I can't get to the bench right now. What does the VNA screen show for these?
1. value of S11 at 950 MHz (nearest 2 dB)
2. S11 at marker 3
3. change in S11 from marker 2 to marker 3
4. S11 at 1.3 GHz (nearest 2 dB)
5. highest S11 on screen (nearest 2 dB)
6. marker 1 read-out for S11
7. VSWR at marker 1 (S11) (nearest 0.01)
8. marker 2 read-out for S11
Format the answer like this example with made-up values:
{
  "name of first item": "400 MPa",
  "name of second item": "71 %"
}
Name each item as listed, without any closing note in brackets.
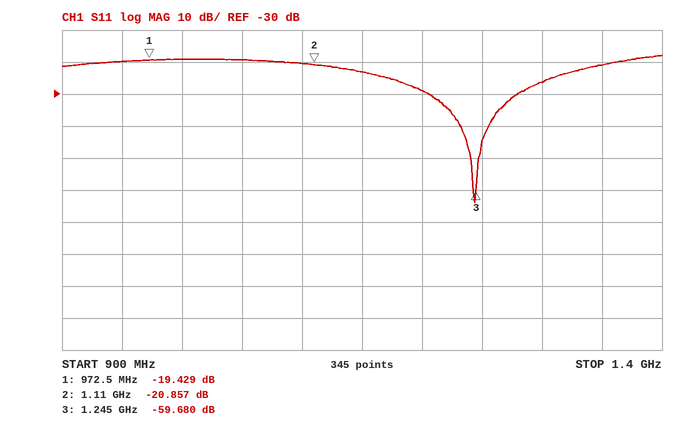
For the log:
{
  "value of S11 at 950 MHz": "-20 dB",
  "S11 at marker 3": "-59.680 dB",
  "change in S11 from marker 2 to marker 3": "-38.823 dB",
  "S11 at 1.3 GHz": "-26 dB",
  "highest S11 on screen": "-18 dB",
  "marker 1 read-out for S11": "-19.429 dB",
  "VSWR at marker 1 (S11)": "1.24",
  "marker 2 read-out for S11": "-20.857 dB"
}
